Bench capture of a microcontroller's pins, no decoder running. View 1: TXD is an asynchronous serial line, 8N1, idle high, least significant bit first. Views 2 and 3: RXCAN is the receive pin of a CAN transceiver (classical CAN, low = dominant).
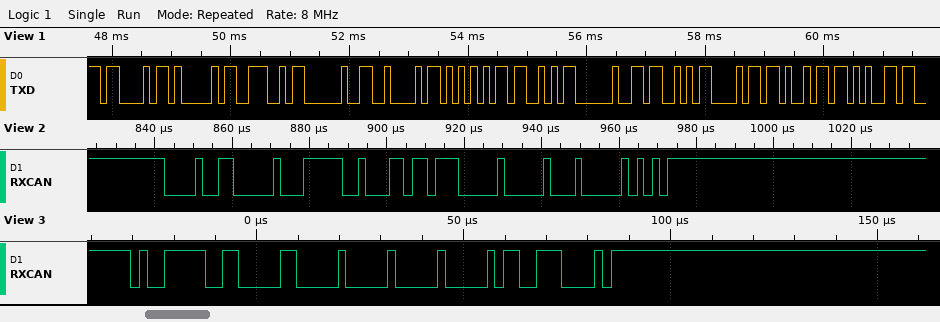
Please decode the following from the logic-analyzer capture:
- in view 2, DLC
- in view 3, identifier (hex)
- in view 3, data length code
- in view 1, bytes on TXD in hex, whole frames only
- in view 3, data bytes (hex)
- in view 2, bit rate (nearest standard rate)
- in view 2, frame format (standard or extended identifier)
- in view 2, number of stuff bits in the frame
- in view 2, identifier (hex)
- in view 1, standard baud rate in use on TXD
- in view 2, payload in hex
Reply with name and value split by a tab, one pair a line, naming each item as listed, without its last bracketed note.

in view 2, DLC	3
in view 3, identifier	0x4FB
in view 3, data length code	2
in view 1, bytes on TXD in hex, whole frames only	43 41 4E 20 42 55 53 20 53 68 69 65
in view 3, data bytes	00 00
in view 2, bit rate	500 kbit/s
in view 2, frame format	standard
in view 2, number of stuff bits in the frame	5
in view 2, identifier	0x098
in view 1, standard baud rate in use on TXD	9600 baud
in view 2, payload in hex	E8 DB 80
